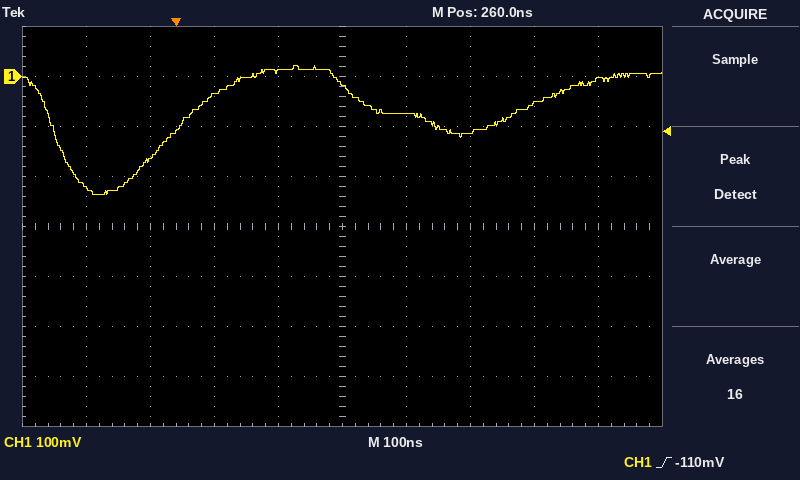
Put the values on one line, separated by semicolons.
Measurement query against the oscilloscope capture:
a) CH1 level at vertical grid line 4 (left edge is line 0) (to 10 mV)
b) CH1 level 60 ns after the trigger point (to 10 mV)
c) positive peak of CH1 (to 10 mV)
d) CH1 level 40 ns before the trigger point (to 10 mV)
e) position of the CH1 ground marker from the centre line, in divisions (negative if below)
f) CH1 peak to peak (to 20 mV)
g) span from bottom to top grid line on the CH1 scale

10 mV; -40 mV; 20 mV; -160 mV; +3.0 div; 260 mV; 800 mV
